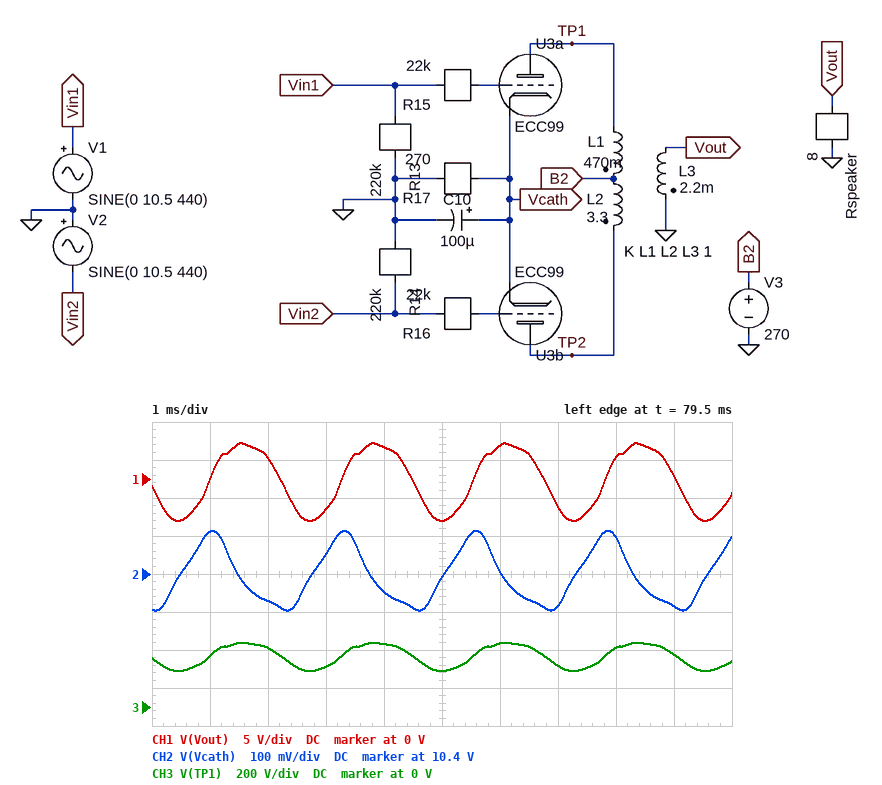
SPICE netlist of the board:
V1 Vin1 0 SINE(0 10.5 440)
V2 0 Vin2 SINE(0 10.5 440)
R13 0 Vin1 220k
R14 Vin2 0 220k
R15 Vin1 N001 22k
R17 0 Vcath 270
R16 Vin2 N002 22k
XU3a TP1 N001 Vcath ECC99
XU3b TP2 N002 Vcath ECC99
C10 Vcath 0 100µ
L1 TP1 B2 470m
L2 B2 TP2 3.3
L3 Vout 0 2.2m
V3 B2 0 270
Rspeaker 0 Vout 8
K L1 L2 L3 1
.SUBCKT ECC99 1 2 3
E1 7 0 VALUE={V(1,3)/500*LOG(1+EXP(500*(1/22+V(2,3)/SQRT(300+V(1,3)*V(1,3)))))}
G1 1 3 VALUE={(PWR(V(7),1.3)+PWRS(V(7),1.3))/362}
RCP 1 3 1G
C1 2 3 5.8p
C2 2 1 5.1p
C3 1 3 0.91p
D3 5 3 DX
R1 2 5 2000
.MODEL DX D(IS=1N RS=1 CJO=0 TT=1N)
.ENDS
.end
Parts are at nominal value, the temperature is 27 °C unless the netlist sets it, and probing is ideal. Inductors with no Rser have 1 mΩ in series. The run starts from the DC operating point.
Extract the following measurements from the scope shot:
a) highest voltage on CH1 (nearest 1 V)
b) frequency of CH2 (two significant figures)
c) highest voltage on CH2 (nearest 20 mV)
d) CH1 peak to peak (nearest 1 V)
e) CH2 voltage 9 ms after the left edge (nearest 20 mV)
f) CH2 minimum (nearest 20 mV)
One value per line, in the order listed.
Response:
5 V
440 Hz
10.52 V
10 V
10.32 V
10.30 V
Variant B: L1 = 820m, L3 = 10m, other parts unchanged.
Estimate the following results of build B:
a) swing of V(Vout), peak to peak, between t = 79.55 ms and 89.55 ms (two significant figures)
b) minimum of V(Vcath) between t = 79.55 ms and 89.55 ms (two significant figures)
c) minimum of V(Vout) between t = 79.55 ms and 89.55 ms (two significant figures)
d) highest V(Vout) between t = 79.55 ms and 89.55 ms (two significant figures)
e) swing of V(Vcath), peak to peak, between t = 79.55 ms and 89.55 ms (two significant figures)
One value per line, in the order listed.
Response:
12 V
11 V
-5.8 V
5.9 V
160 mV
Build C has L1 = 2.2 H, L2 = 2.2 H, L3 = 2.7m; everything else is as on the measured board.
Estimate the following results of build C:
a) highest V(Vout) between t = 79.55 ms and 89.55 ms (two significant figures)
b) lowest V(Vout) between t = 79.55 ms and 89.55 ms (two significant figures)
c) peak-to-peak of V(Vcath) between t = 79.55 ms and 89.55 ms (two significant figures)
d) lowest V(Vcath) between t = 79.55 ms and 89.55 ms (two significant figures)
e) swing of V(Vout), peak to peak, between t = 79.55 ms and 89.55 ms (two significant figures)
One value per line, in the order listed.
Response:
5.8 V
-5.8 V
21 mV
9.5 V
12 V
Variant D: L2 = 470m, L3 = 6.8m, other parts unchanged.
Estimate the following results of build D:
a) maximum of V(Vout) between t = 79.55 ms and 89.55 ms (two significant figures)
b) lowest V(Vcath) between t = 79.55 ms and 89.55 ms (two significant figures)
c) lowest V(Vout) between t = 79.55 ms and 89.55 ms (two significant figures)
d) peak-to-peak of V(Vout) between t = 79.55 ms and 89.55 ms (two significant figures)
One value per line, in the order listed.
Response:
4.6 V
12 V
-4.6 V
9.2 V
